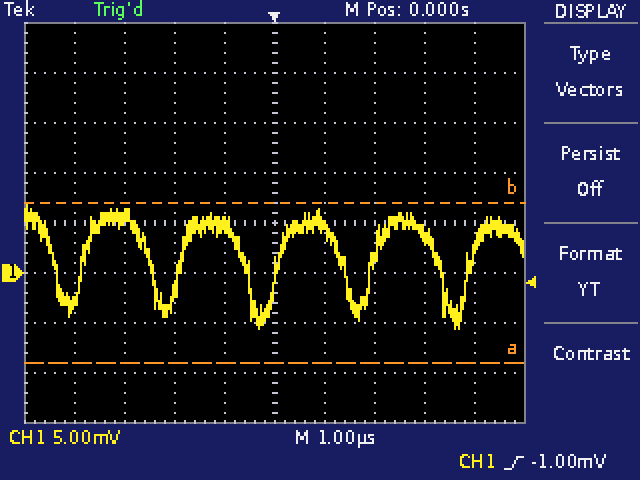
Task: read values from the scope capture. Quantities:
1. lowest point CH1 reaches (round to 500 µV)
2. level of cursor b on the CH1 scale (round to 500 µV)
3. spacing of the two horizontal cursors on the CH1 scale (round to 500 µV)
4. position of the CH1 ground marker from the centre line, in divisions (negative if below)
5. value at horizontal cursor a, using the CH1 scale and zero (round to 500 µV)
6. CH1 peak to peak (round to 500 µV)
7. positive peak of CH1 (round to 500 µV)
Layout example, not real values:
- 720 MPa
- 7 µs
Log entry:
- -5.5 mV
- 7.0 mV
- 16.0 mV
- -1.0 div
- -9.0 mV
- 12.5 mV
- 7.0 mV
